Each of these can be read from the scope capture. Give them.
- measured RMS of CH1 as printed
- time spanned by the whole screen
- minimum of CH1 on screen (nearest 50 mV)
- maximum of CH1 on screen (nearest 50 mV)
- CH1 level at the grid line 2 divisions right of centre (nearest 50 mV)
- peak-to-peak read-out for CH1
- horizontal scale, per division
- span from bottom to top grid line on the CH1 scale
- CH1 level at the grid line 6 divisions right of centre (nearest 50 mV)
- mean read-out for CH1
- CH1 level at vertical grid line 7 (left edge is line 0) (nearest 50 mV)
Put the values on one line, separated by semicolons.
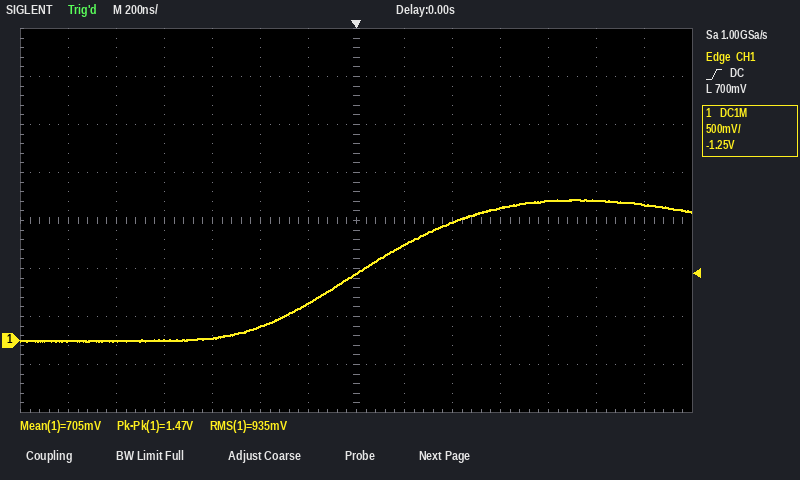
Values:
935 mV; 2.8 µs; 0 mV; 1.45 V; 1.25 V; 1.47 V; 200 ns; 4 V; 1.40 V; 705 mV; 700 mV
